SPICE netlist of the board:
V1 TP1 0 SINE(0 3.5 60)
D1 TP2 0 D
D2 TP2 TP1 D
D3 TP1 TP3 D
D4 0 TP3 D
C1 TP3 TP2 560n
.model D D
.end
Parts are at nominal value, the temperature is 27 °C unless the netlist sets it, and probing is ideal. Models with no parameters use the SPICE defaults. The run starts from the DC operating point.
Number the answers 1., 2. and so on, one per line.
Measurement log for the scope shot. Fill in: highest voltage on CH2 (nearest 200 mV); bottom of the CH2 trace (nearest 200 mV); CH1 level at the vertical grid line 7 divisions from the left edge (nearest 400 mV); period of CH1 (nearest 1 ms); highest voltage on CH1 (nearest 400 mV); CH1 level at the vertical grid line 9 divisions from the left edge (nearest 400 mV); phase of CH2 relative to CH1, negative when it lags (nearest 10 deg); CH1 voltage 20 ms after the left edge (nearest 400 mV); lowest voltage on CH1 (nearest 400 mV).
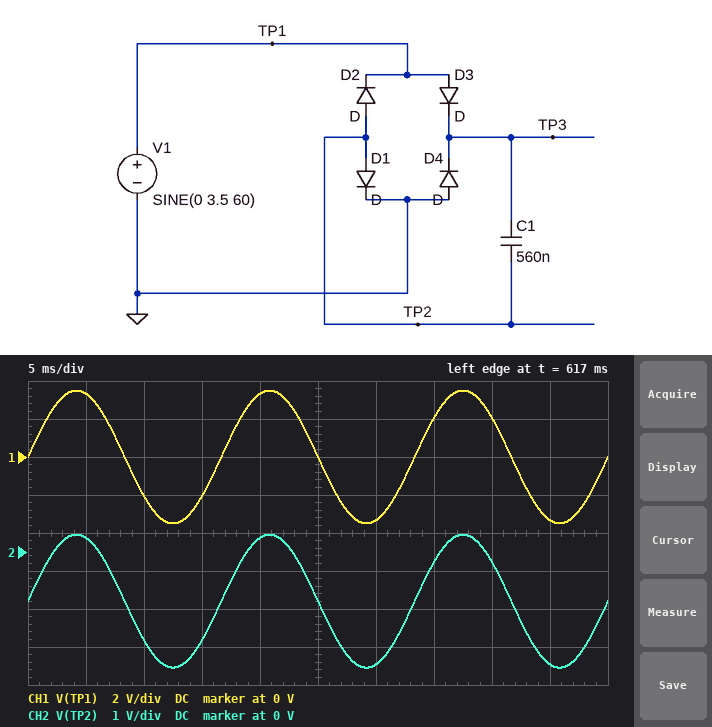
1. 400 mV
2. -3.0 V
3. 2.0 V
4. 17 ms
5. 3.6 V
6. -3.2 V
7. 0 deg
8. 3.2 V
9. -3.6 V
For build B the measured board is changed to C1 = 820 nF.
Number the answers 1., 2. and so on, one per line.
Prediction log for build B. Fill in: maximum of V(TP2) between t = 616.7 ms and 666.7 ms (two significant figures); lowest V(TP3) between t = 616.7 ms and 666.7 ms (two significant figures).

1. 470 mV
2. -470 mV
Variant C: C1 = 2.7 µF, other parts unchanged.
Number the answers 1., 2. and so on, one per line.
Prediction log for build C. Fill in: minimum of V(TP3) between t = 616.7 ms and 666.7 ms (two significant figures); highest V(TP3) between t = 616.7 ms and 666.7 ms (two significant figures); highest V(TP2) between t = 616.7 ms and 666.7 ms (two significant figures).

1. -500 mV
2. 3.0 V
3. 500 mV
